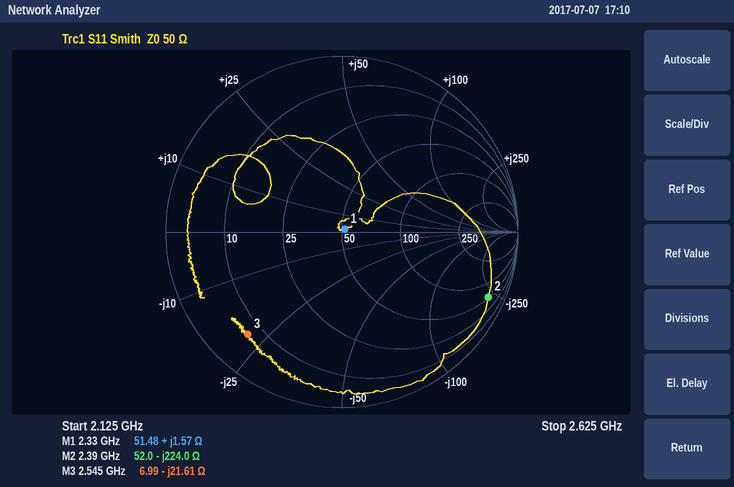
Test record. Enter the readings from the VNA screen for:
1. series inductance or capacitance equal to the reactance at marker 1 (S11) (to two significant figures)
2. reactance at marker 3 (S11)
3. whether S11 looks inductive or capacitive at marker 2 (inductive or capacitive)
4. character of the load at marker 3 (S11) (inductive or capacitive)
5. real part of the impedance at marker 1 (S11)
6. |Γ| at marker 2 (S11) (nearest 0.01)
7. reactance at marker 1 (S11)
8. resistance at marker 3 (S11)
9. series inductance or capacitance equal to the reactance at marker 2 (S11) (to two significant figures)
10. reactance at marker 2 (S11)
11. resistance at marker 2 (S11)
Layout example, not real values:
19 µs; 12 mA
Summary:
110 pH; -21.61 Ω; capacitive; capacitive; 51.48 Ω; 0.91; +1.57 Ω; 6.99 Ω; 300 fF; -224.0 Ω; 52.0 Ω
